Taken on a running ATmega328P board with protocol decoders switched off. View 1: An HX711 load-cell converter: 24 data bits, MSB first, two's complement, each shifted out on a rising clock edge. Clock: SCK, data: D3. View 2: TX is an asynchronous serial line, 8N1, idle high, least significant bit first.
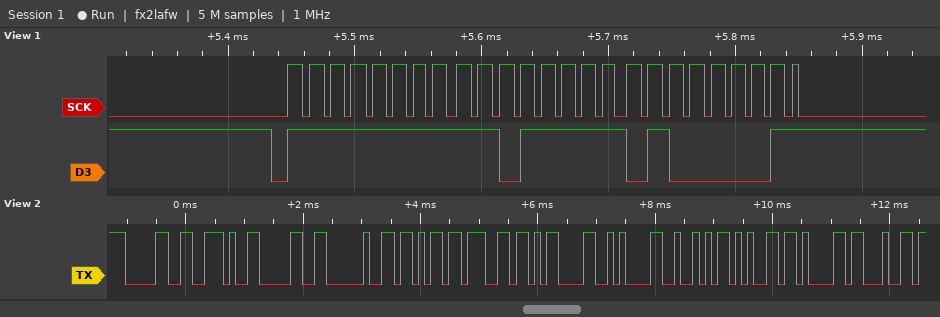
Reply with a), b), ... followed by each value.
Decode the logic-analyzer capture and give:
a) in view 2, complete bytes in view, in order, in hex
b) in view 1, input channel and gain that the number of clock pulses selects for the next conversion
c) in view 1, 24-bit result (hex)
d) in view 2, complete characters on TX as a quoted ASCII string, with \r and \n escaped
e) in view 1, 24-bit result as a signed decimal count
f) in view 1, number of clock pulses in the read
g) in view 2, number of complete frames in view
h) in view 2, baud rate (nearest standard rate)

a) 30 2E 30 20 6B 67 0D 0A 52 65 61 64
b) channel A, gain 128
c) 0xFFDF41
d) "0.0 kg\r\nRead"
e) -8383
f) 25
g) 12
h) 9600 baud
